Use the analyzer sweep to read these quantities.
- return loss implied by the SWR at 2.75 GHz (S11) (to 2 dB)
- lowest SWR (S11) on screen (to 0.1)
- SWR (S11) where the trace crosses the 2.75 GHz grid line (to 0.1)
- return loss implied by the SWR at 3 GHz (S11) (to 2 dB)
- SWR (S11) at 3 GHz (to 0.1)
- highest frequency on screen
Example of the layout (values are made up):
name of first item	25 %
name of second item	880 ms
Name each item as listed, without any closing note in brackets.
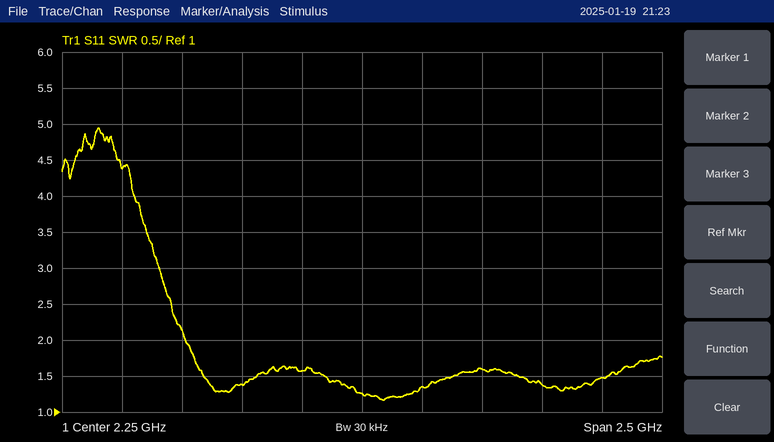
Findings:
return loss implied by the SWR at 2.75 GHz (S11)	12 dB
lowest SWR (S11) on screen	1.2
SWR (S11) where the trace crosses the 2.75 GHz grid line	1.6
return loss implied by the SWR at 3 GHz (S11)	16 dB
SWR (S11) at 3 GHz	1.4
highest frequency on screen	3.5 GHz
